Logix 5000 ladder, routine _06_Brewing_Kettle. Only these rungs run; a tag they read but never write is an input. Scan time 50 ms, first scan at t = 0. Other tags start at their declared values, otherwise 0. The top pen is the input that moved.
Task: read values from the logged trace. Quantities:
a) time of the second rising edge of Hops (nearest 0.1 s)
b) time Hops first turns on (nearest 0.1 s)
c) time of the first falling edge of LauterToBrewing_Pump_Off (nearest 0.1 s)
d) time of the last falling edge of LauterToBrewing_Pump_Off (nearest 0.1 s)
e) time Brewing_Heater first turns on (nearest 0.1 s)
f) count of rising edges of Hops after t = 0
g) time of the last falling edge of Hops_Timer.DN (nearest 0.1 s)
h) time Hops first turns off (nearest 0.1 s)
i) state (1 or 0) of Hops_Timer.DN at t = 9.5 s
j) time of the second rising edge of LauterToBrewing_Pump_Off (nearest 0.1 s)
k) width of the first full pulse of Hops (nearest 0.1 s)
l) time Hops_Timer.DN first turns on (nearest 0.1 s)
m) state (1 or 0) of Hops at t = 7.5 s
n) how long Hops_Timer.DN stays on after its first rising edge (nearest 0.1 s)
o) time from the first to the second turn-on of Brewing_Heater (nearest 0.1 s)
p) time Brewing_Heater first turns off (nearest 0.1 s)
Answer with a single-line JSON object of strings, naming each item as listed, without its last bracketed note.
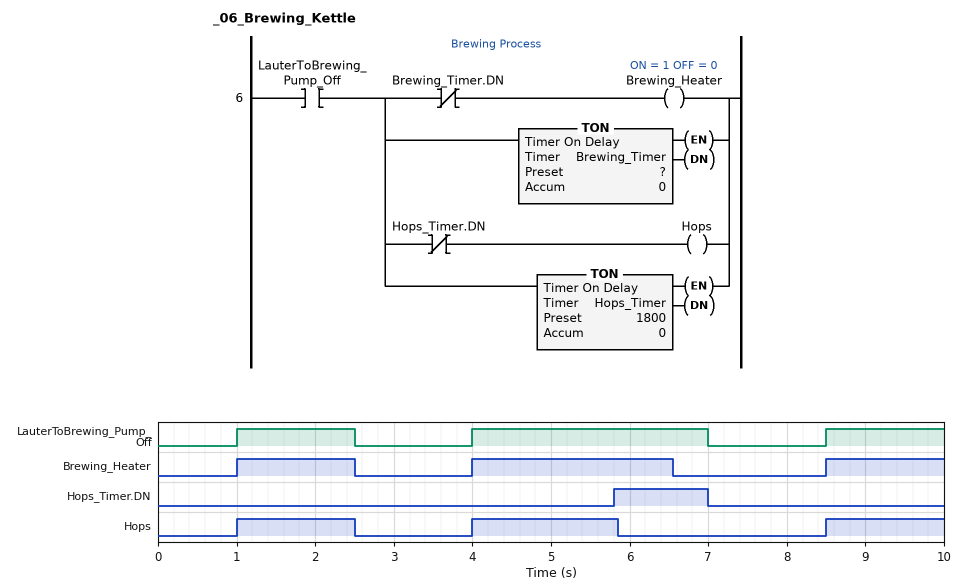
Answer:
{"time of the second rising edge of Hops": "4.0 s", "time Hops first turns on": "1.0 s", "time of the first falling edge of LauterToBrewing_Pump_Off": "2.5 s", "time of the last falling edge of LauterToBrewing_Pump_Off": "7.0 s", "time Brewing_Heater first turns on": "1.0 s", "count of rising edges of Hops after t = 0": "3", "time of the last falling edge of Hops_Timer.DN": "7.0 s", "time Hops first turns off": "2.5 s", "state (1 or 0) of Hops_Timer.DN at t = 9.5 s": "0", "time of the second rising edge of LauterToBrewing_Pump_Off": "4.0 s", "width of the first full pulse of Hops": "1.5 s", "time Hops_Timer.DN first turns on": "5.8 s", "state (1 or 0) of Hops at t = 7.5 s": "0", "how long Hops_Timer.DN stays on after its first rising edge": "1.2 s", "time from the first to the second turn-on of Brewing_Heater": "3.0 s", "time Brewing_Heater first turns off": "2.5 s"}
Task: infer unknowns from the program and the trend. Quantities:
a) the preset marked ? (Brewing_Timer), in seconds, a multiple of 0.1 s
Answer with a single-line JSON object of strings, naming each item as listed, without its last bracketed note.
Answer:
{"the preset marked ? (Brewing_Timer), in seconds, a multiple of 0.1 s": "2.5 s"}
